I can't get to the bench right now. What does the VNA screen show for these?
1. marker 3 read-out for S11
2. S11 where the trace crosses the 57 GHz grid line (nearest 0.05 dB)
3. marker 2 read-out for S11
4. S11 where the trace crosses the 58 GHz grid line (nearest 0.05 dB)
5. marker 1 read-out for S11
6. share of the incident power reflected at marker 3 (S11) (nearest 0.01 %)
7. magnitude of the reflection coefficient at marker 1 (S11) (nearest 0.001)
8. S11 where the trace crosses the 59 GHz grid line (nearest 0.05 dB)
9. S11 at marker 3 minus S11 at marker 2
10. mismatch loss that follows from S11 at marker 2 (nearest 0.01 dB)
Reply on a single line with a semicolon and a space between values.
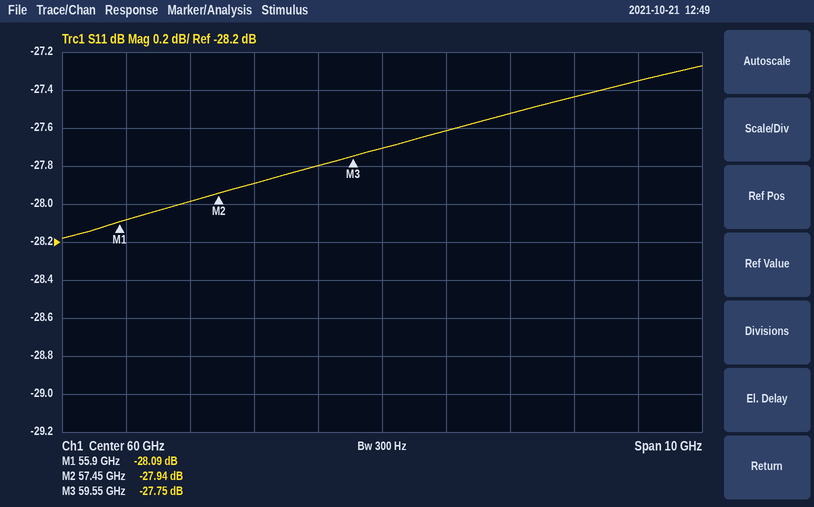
-27.75 dB; -28.00 dB; -27.94 dB; -27.90 dB; -28.09 dB; 0.17 %; 0.039; -27.80 dB; 0.19 dB; 0.01 dB
